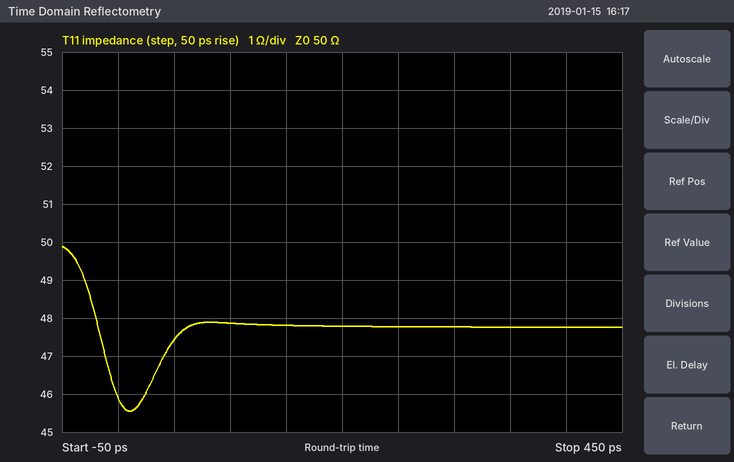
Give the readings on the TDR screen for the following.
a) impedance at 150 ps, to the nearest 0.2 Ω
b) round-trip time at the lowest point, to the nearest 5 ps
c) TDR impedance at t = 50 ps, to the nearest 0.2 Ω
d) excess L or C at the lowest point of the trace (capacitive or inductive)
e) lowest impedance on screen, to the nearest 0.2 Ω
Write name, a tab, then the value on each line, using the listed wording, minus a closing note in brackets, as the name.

impedance at 150 ps, to the nearest 0.2 Ω	47.8 Ω
round-trip time at the lowest point, to the nearest 5 ps	10 ps
TDR impedance at t = 50 ps, to the nearest 0.2 Ω	47.4 Ω
excess L or C at the lowest point of the trace	capacitive
lowest impedance on screen, to the nearest 0.2 Ω	45.6 Ω
